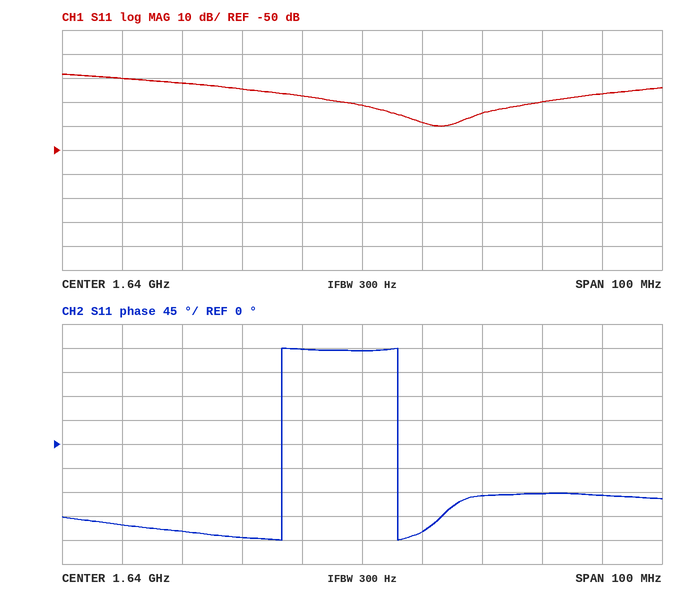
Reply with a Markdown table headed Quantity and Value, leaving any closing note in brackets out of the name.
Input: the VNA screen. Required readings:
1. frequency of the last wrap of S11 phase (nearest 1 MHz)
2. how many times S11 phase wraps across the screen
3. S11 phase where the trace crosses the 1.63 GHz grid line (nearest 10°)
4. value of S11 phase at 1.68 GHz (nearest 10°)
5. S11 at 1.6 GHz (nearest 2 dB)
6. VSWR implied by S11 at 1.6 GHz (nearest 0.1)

| Quantity | Value |
|---|---|
| frequency of the last wrap of S11 phase | 1.646 GHz |
| how many times S11 phase wraps across the screen | 2 |
| S11 phase where the trace crosses the 1.63 GHz grid line | 180° |
| value of S11 phase at 1.68 GHz | -100° |
| S11 at 1.6 GHz | -20 dB |
| VSWR implied by S11 at 1.6 GHz | 1.2 |
